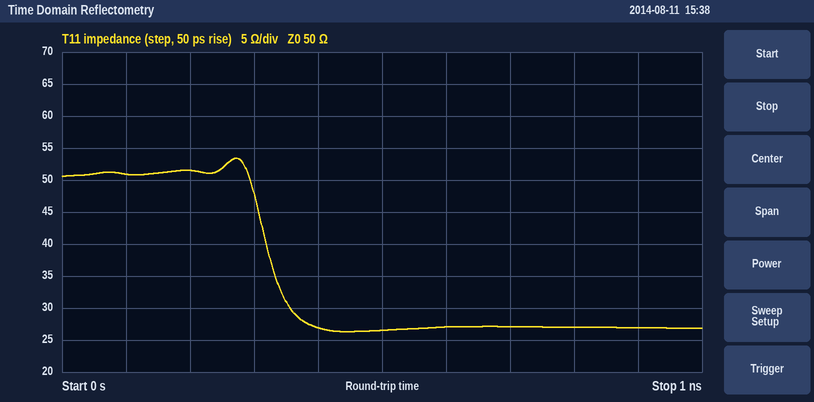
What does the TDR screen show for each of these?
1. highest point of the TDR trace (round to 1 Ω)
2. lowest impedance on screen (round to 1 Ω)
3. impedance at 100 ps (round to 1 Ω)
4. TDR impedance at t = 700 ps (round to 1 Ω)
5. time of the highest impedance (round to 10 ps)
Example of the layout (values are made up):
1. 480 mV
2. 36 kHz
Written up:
1. 53 Ω
2. 26 Ω
3. 51 Ω
4. 27 Ω
5. 270 ps
